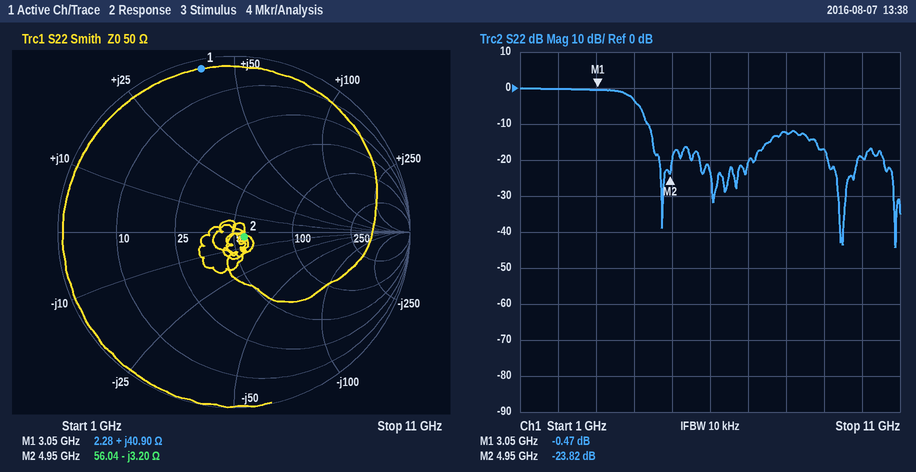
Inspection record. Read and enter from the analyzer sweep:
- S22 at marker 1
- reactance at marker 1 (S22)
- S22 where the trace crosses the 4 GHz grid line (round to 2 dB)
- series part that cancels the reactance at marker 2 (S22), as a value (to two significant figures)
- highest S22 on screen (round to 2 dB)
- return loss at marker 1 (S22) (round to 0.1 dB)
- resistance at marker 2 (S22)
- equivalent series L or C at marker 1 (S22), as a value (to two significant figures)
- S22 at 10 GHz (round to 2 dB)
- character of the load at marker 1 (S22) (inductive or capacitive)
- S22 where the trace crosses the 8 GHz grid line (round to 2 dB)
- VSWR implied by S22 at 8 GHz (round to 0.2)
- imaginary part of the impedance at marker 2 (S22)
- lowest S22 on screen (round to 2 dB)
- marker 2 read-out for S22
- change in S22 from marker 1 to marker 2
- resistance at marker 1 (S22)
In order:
-0.47 dB
+40.90 Ω
-4 dB
100 pH
0 dB
0.5 dB
56.04 Ω
2.1 nH
-20 dB
inductive
-12 dB
1.6
-3.20 Ω
-44 dB
-23.82 dB
-23.35 dB
2.28 Ω
